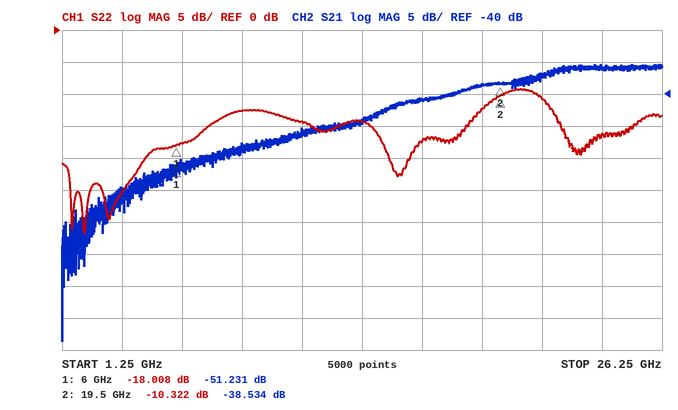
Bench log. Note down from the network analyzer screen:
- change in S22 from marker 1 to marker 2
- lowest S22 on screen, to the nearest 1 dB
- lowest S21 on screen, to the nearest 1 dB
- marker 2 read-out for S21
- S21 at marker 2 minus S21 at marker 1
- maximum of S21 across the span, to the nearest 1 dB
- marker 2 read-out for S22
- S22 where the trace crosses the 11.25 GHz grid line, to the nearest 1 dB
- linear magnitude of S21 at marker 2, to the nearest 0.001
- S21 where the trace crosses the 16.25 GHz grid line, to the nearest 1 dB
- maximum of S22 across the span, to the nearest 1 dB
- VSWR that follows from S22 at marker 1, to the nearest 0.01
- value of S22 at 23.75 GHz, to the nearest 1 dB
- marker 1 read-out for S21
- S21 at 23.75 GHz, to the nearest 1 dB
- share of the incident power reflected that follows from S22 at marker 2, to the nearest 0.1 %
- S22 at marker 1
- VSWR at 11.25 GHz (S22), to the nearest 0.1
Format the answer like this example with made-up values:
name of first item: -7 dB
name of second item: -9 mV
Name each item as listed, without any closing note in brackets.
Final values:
change in S22 from marker 1 to marker 2: 7.686 dB
lowest S22 on screen, to the nearest 1 dB: -32 dB
lowest S21 on screen, to the nearest 1 dB: -79 dB
marker 2 read-out for S21: -38.534 dB
S21 at marker 2 minus S21 at marker 1: 12.697 dB
maximum of S21 across the span, to the nearest 1 dB: -35 dB
marker 2 read-out for S22: -10.322 dB
S22 where the trace crosses the 11.25 GHz grid line, to the nearest 1 dB: -14 dB
linear magnitude of S21 at marker 2, to the nearest 0.001: 0.012
S21 where the trace crosses the 16.25 GHz grid line, to the nearest 1 dB: -41 dB
maximum of S22 across the span, to the nearest 1 dB: -9 dB
VSWR that follows from S22 at marker 1, to the nearest 0.01: 1.29
value of S22 at 23.75 GHz, to the nearest 1 dB: -16 dB
marker 1 read-out for S21: -51.231 dB
S21 at 23.75 GHz, to the nearest 1 dB: -36 dB
share of the incident power reflected that follows from S22 at marker 2, to the nearest 0.1 %: 9.3 %
S22 at marker 1: -18.008 dB
VSWR at 11.25 GHz (S22), to the nearest 0.1: 1.5
